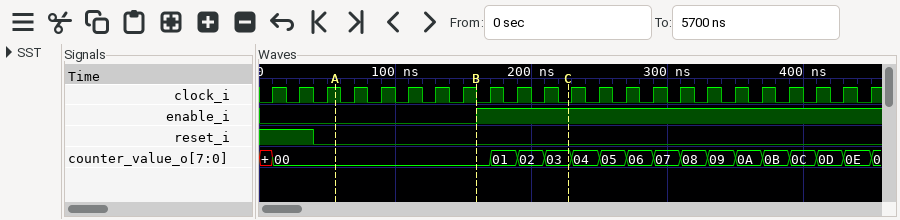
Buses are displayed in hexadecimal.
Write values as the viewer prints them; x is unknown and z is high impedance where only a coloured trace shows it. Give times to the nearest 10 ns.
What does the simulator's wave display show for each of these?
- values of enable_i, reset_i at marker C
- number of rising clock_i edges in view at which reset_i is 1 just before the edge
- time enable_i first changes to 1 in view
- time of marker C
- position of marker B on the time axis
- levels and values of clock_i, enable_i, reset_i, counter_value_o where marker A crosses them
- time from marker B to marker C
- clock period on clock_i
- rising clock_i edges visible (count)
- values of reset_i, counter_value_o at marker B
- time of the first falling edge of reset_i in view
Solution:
enable_i=1, reset_i=0
2
160 ns
230 ns
160 ns
clock_i=1, enable_i=0, reset_i=0, counter_value_o=00
70 ns
20 ns
23
reset_i=0, counter_value_o=00
40 ns
